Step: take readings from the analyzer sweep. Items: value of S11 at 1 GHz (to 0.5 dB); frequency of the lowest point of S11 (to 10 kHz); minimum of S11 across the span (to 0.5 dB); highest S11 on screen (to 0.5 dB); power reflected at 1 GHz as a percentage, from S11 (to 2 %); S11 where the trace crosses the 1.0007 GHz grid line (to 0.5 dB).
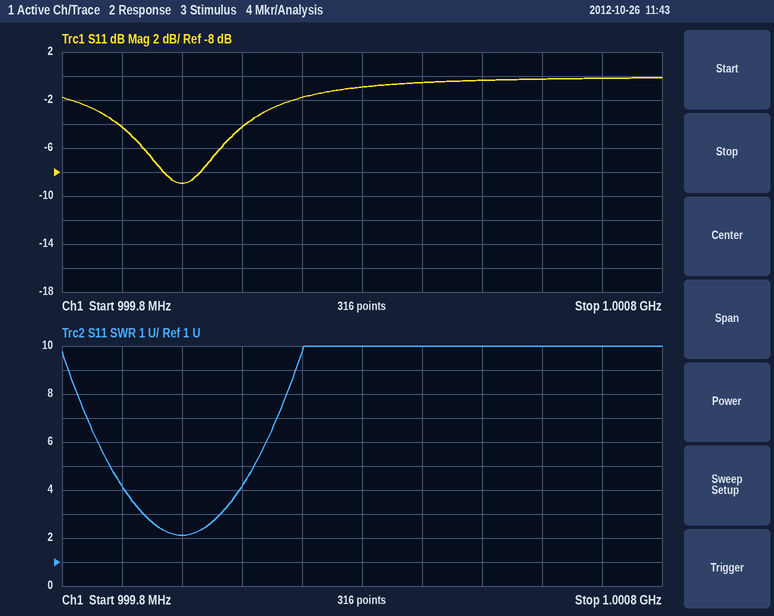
-9.0 dB
1.00000 GHz
-9.0 dB
0.0 dB
12 %
0.0 dB
